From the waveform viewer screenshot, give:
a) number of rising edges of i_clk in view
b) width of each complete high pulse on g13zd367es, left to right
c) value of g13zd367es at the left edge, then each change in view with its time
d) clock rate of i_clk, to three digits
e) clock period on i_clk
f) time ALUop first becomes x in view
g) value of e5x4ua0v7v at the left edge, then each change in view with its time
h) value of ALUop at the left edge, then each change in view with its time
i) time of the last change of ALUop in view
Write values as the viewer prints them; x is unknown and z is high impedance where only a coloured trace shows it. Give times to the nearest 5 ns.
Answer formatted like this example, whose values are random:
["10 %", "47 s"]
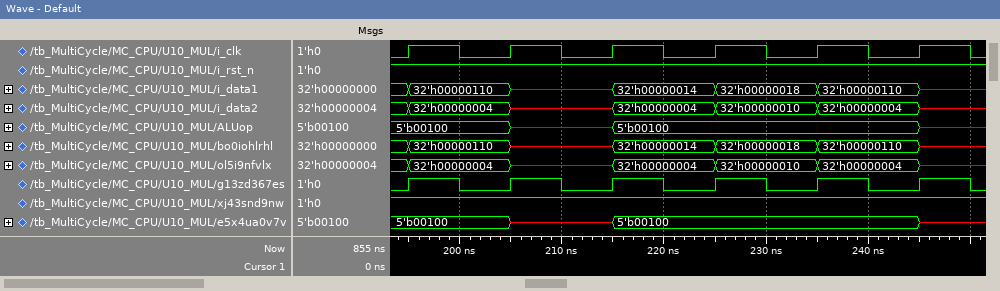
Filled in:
["6", "5 ns, 5 ns, 5 ns, 5 ns, 5 ns, 5 ns", "0, 1 at 195 ns, 0 at 200 ns, 1 at 205 ns, 0 at 210 ns, 1 at 215 ns, 0 at 220 ns, 1 at 225 ns, 0 at 230 ns, 1 at 235 ns, 0 at 240 ns, 1 at 245 ns, 0 at 250 ns", "100 MHz", "10 ns", "205 ns", "5'b00100, x at 205 ns, 5'b00100 at 215 ns, x at 245 ns", "5'b00100, x at 205 ns, 5'b00100 at 215 ns, x at 245 ns", "245 ns"]
